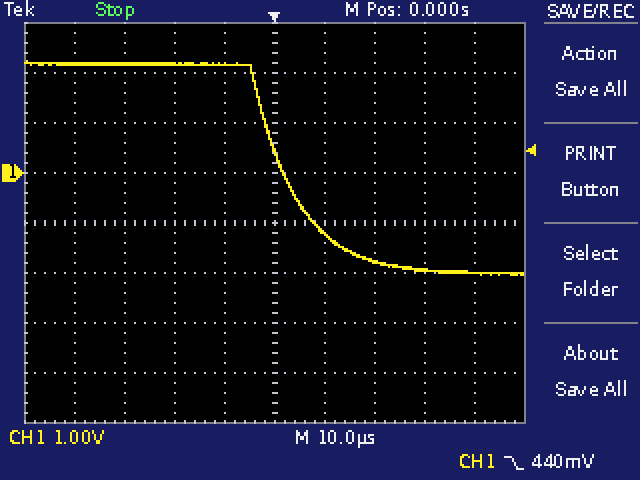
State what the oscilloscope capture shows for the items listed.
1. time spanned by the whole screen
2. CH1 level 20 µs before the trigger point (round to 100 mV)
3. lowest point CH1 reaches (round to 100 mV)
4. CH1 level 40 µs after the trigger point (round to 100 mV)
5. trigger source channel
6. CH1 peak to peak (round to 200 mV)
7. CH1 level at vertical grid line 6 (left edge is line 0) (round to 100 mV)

100 µs
2.2 V
-2.0 V
-2.0 V
CH1
4.2 V
-1.2 V
